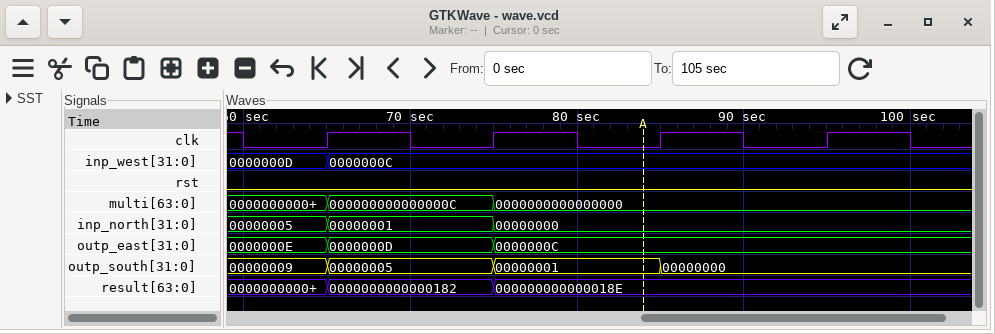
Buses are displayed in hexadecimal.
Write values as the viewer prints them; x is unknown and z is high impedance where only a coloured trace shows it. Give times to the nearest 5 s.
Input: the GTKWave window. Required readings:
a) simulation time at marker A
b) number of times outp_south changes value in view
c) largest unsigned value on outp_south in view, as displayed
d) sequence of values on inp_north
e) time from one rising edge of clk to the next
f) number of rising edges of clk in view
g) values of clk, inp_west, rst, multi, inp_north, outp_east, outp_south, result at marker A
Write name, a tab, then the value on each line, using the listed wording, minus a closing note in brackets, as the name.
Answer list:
simulation time at marker A	85 s
number of times outp_south changes value in view	3
largest unsigned value on outp_south in view, as displayed	00000009
sequence of values on inp_north	00000005, 00000001, 00000000
time from one rising edge of clk to the next	10 s
number of rising edges of clk in view	4
values of clk, inp_west, rst, multi, inp_north, outp_east, outp_south, result at marker A	clk=0, inp_west=0000000C, rst=0, multi=0000000000000000, inp_north=00000000, outp_east=0000000C, outp_south=00000001, result=000000000000018E
